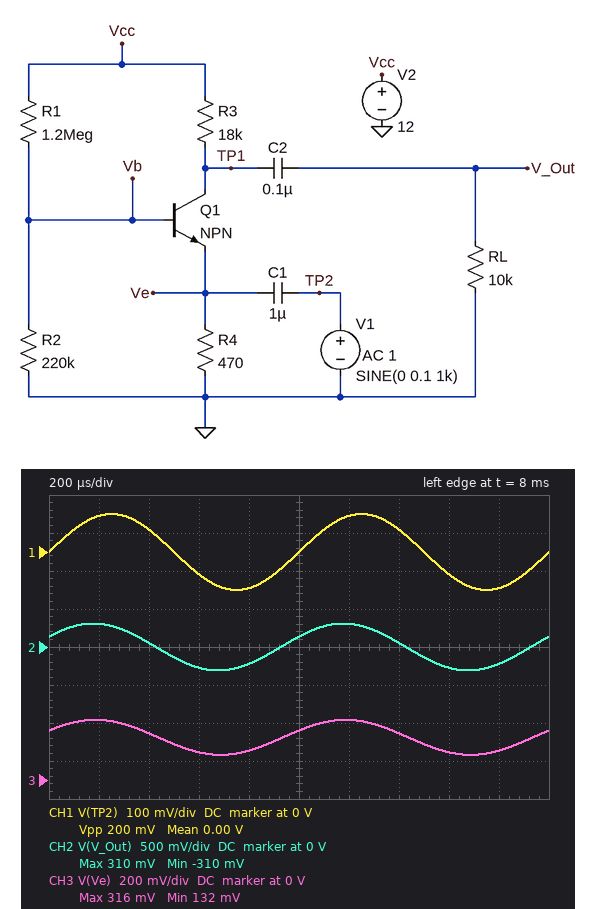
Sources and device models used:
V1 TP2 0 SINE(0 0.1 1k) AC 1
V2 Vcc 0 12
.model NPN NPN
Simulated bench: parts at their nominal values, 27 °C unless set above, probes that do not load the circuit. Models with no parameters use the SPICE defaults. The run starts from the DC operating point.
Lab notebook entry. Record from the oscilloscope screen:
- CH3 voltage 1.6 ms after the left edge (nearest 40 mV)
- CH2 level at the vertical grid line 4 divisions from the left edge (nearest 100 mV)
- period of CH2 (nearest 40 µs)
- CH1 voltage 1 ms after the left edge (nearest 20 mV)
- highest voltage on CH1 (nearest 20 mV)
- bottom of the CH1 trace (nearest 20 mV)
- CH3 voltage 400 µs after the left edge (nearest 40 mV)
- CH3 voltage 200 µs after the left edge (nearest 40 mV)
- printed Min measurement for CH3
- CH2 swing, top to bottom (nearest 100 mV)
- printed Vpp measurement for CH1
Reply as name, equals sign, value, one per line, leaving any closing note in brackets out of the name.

CH3 voltage 1.6 ms after the left edge = 160 mV
CH2 level at the vertical grid line 4 divisions from the left edge = -200 mV
period of CH2 = 1.00 ms
CH1 voltage 1 ms after the left edge = 0 V
highest voltage on CH1 = 100 mV
bottom of the CH1 trace = -100 mV
CH3 voltage 400 µs after the left edge = 240 mV
CH3 voltage 200 µs after the left edge = 320 mV
printed Min measurement for CH3 = 132 mV
CH2 swing, top to bottom = 600 mV
printed Vpp measurement for CH1 = 200 mV
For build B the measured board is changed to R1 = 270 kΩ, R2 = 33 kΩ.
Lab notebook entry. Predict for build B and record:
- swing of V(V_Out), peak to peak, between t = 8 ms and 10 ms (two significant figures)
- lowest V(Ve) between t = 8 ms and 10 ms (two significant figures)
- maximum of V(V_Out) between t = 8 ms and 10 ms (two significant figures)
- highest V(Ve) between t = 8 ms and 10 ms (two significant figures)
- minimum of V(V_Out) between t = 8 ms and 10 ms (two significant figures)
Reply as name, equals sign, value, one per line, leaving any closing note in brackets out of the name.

swing of V(V_Out), peak to peak, between t = 8 ms and 10 ms = 890 mV
lowest V(Ve) between t = 8 ms and 10 ms = 210 mV
maximum of V(V_Out) between t = 8 ms and 10 ms = 640 mV
highest V(Ve) between t = 8 ms and 10 ms = 390 mV
minimum of V(V_Out) between t = 8 ms and 10 ms = -250 mV
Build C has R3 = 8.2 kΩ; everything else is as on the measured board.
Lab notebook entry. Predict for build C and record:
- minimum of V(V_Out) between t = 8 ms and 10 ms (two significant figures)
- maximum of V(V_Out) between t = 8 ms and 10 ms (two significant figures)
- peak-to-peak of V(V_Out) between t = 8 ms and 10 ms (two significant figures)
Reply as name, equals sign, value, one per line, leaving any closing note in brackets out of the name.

minimum of V(V_Out) between t = 8 ms and 10 ms = -220 mV
maximum of V(V_Out) between t = 8 ms and 10 ms = 220 mV
peak-to-peak of V(V_Out) between t = 8 ms and 10 ms = 430 mV
